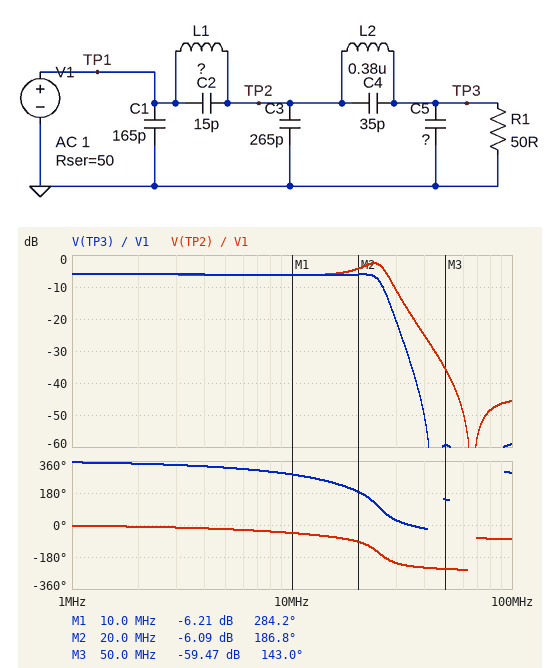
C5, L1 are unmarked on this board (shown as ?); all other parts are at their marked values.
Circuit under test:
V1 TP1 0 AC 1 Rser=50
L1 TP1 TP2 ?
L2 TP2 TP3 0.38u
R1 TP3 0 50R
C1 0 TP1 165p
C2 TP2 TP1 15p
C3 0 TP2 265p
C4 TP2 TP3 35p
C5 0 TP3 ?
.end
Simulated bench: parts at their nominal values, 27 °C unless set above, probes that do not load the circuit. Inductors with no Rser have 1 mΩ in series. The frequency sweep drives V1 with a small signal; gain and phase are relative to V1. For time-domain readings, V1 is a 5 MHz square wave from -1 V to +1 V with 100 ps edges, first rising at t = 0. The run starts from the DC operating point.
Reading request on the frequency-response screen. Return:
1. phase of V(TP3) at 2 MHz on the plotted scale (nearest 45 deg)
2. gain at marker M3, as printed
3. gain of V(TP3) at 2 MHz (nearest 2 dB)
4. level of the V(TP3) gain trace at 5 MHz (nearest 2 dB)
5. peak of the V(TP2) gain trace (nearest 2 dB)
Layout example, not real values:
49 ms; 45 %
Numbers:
360 deg; -59.47 dB; -6 dB; -6 dB; -2 dB
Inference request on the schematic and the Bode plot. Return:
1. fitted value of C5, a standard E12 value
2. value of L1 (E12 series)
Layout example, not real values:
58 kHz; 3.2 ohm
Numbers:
100 pF; 390 nH
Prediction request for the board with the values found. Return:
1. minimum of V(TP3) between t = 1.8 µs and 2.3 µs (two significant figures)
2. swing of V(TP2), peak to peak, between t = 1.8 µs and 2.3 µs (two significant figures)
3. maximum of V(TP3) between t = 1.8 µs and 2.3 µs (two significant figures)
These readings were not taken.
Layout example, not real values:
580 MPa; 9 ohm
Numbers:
-680 mV; 1.4 V; 680 mV
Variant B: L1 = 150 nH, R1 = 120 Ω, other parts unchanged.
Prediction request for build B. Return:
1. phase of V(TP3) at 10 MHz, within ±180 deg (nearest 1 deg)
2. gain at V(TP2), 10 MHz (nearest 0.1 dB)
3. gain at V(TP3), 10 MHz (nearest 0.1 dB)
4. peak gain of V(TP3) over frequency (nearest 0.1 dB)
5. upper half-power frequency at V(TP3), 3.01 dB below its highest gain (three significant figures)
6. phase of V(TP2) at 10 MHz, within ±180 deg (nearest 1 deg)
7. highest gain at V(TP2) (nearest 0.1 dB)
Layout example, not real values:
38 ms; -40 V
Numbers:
-65 deg; -6.2 dB; -5.0 dB; -3.0 dB; 26.1 MHz; -51 deg; -2.4 dB
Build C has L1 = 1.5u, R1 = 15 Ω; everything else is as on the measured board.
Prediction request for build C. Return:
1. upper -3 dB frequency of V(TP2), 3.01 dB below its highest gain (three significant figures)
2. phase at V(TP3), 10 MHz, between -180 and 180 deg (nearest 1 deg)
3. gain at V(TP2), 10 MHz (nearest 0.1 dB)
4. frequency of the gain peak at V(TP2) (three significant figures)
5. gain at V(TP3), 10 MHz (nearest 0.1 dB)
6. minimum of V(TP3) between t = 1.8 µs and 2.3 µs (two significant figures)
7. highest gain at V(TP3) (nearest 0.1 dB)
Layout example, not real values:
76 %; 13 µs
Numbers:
18.0 MHz; -111 deg; -10.7 dB; 16.2 MHz; -16.2 dB; -240 mV; -12.7 dB
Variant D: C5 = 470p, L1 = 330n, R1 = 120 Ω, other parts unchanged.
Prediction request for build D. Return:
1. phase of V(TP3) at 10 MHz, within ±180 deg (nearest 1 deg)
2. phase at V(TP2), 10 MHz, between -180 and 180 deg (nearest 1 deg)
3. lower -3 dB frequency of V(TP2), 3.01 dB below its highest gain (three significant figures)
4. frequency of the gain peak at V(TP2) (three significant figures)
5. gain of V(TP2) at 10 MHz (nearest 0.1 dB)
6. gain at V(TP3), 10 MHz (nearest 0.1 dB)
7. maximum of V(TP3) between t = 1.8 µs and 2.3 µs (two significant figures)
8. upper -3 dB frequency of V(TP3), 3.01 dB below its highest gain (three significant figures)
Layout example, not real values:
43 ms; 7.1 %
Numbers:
-102 deg; -63 deg; 20.2 MHz; 24.4 MHz; -14.7 dB; -5.1 dB; 690 mV; 15.7 MHz
